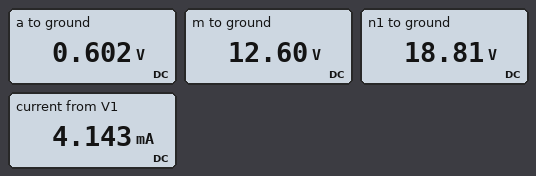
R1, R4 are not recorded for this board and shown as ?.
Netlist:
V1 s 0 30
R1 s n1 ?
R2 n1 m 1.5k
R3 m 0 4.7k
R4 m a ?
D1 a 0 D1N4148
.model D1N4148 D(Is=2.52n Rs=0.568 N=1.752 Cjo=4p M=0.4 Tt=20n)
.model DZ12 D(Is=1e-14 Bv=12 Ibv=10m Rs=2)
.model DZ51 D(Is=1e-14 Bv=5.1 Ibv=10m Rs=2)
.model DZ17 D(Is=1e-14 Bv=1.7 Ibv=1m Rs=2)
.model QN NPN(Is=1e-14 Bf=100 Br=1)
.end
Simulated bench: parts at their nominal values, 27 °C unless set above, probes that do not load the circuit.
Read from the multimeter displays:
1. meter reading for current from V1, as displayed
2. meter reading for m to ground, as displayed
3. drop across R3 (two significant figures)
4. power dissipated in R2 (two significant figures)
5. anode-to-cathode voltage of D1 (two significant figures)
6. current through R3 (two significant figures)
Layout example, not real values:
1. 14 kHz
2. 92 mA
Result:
1. 4.143 mA
2. 12.60 V
3. 13 V
4. 26 mW
5. 600 mV
6. 2.7 mA
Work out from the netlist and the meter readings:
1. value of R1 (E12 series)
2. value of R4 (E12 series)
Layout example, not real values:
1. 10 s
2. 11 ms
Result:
1. 2.7 kΩ
2. 8.2 kΩ
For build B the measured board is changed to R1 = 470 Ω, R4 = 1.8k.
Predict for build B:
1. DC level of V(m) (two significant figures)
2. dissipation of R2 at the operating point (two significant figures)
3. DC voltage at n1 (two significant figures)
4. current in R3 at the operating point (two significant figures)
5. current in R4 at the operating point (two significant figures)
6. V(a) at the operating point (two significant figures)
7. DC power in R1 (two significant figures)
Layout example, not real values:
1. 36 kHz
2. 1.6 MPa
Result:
1. 12 V
2. 120 mW
3. 26 V
4. 2.6 mA
5. 6.4 mA
6. 670 mV
7. 38 mW
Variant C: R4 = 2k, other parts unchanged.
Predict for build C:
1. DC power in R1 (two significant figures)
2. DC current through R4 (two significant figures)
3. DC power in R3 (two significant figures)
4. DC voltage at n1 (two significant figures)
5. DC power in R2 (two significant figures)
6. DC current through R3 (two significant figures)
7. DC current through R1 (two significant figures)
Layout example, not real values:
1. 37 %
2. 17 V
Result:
1. 75 mW
2. 3.6 mA
3. 13 mW
4. 16 V
5. 42 mW
6. 1.7 mA
7. 5.3 mA
